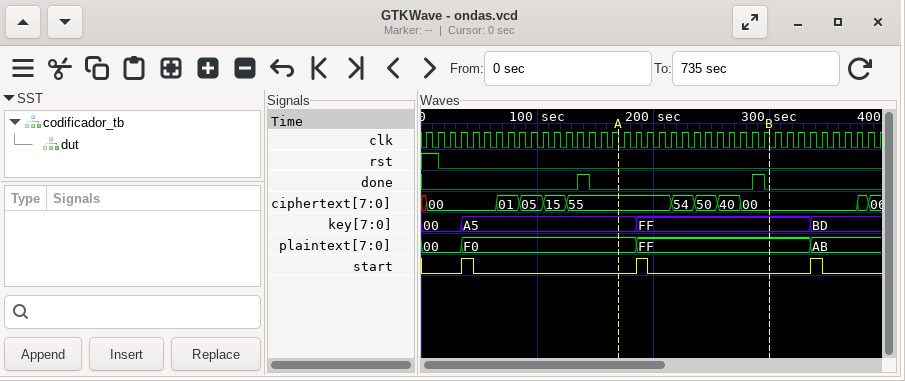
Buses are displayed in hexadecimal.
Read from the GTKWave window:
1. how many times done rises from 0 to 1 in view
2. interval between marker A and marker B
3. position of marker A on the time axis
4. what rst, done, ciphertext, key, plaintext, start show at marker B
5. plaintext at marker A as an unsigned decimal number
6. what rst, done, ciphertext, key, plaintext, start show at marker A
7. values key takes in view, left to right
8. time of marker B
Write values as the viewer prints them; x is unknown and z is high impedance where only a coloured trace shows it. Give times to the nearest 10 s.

2
130 s
170 s
rst=0, done=0, ciphertext=00, key=FF, plaintext=FF, start=0
240
rst=0, done=0, ciphertext=55, key=A5, plaintext=F0, start=0
00, A5, FF, BD
300 s
